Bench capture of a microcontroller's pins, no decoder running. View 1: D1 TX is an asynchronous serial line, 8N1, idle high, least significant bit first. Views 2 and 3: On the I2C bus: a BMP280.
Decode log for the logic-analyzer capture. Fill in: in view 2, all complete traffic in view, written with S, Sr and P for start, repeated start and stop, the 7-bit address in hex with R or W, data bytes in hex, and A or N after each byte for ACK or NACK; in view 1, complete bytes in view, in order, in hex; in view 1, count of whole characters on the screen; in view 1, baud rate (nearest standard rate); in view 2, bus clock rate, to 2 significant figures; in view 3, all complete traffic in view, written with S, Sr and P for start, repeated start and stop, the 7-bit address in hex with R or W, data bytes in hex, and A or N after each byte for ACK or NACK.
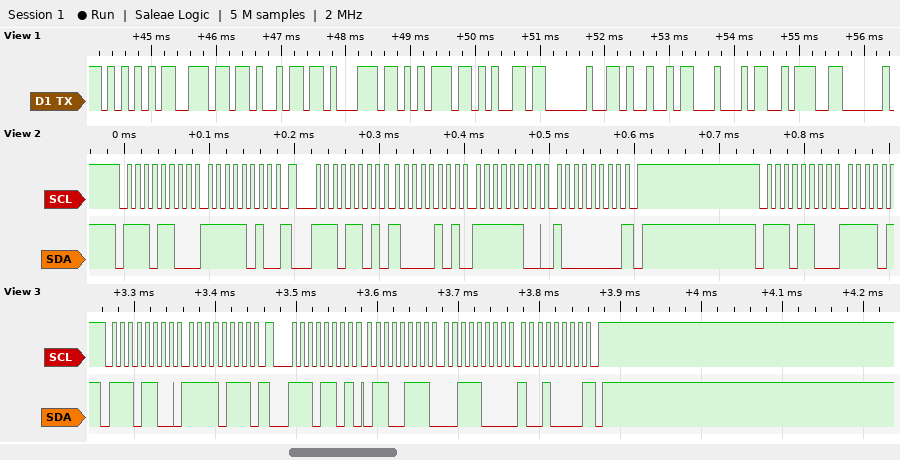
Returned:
S 76W A FA A Sr 76R A 85 A FC A 80 N P S 76W A
55 6E 69 71 75 65 20 49 44 3A
10
9600 baud
100 kHz
S 76W A F7 A Sr 76R A 67 A 38 A 90 N P
